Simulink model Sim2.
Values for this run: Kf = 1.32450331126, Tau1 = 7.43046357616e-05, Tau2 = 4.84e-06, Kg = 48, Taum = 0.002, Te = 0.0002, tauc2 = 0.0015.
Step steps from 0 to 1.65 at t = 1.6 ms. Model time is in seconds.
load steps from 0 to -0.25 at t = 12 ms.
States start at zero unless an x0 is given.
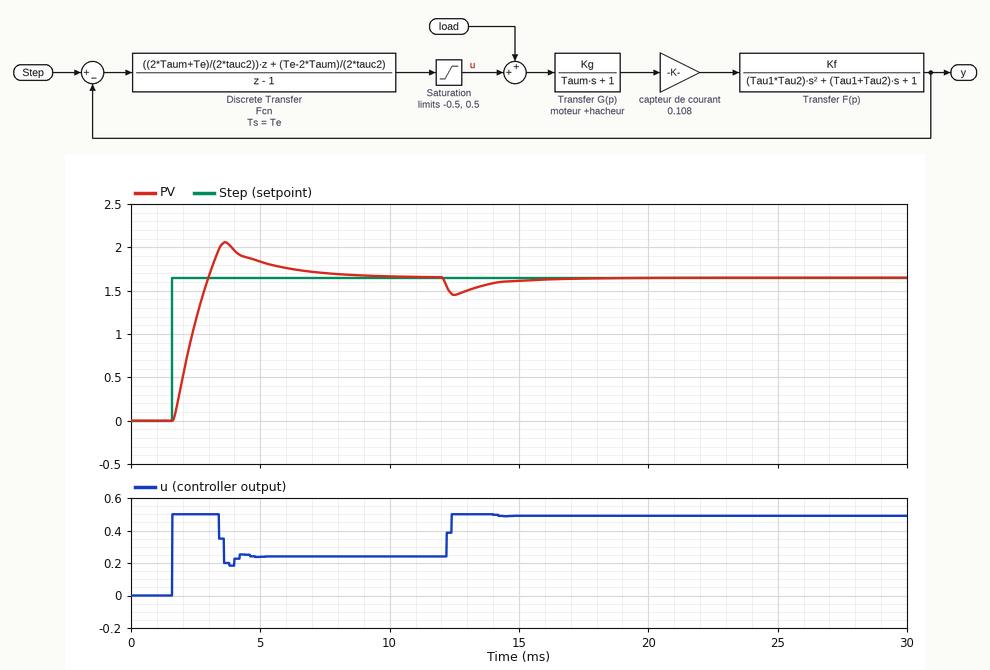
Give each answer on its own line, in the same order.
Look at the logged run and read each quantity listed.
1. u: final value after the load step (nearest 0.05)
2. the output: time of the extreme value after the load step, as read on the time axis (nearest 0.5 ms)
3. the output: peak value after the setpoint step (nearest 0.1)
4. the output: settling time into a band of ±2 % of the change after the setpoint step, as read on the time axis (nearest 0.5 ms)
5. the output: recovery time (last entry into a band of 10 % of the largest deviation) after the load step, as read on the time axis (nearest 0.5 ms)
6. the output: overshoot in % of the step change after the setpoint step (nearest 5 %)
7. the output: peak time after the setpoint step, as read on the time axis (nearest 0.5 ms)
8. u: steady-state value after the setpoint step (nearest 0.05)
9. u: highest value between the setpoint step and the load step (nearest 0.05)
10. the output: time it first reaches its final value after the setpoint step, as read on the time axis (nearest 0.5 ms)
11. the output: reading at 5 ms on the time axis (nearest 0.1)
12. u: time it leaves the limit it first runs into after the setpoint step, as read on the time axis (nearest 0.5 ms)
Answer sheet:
0.50
12.5 ms
2.1
8.5 ms
16.0 ms
25 %
3.5 ms
0.25
0.50
3.0 ms
1.8
3.5 ms
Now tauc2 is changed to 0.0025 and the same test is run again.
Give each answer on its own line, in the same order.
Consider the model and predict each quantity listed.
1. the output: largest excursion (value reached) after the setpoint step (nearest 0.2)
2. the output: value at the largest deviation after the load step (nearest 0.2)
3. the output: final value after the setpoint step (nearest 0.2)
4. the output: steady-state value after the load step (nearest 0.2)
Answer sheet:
2.0
1.4
1.6
1.6
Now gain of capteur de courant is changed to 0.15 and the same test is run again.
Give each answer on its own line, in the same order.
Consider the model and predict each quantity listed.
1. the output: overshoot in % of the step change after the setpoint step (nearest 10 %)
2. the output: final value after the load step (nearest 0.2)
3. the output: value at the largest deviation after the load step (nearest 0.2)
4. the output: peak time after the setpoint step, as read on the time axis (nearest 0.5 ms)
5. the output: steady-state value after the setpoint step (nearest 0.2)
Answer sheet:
30 %
1.6
1.4
3.0 ms
1.6
